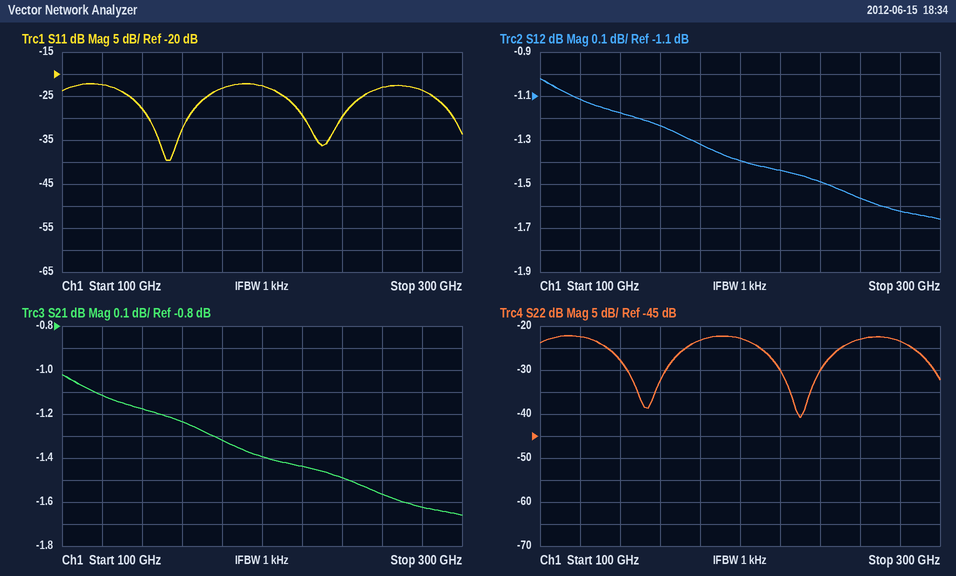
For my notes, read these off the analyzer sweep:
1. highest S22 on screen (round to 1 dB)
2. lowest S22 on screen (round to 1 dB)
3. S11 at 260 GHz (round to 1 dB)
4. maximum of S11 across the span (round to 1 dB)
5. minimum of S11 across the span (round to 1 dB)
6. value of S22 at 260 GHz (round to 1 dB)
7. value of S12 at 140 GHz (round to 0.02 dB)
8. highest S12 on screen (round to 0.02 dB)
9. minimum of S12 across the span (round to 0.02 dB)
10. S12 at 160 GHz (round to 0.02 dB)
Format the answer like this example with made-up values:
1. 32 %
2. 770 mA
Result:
1. -22 dB
2. -41 dB
3. -23 dB
4. -22 dB
5. -40 dB
6. -23 dB
7. -1.18 dB
8. -1.02 dB
9. -1.66 dB
10. -1.24 dB
